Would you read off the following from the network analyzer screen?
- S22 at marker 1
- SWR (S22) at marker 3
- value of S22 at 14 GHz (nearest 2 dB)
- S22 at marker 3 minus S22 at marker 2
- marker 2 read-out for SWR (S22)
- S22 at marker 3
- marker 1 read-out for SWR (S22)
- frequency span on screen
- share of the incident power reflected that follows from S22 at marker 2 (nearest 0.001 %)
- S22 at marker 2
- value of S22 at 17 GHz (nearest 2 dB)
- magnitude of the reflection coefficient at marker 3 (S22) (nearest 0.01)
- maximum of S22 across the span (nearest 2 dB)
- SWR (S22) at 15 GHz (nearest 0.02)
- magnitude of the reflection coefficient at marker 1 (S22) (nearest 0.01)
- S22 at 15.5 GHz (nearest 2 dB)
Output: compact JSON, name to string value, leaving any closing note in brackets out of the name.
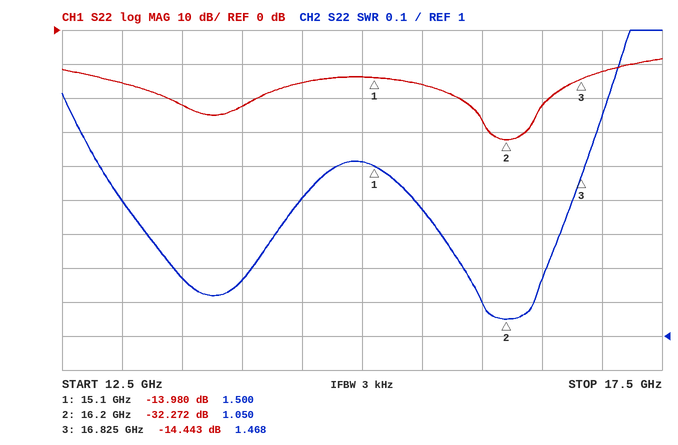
{"S22 at marker 1": "-13.980 dB", "SWR (S22) at marker 3": "1.468", "value of S22 at 14 GHz": "-22 dB", "S22 at marker 3 minus S22 at marker 2": "17.829 dB", "marker 2 read-out for SWR": "1.050", "S22 at marker 3": "-14.443 dB", "marker 1 read-out for SWR": "1.500", "frequency span on screen": "5 GHz", "share of the incident power reflected that follows from S22 at marker 2": "0.059 %", "S22 at marker 2": "-32.272 dB", "value of S22 at 17 GHz": "-12 dB", "magnitude of the reflection coefficient at marker 3 (S22)": "0.19", "maximum of S22 across the span": "-8 dB", "SWR (S22) at 15 GHz": "1.52", "magnitude of the reflection coefficient at marker 1 (S22)": "0.20", "S22 at 15.5 GHz": "-16 dB"}
